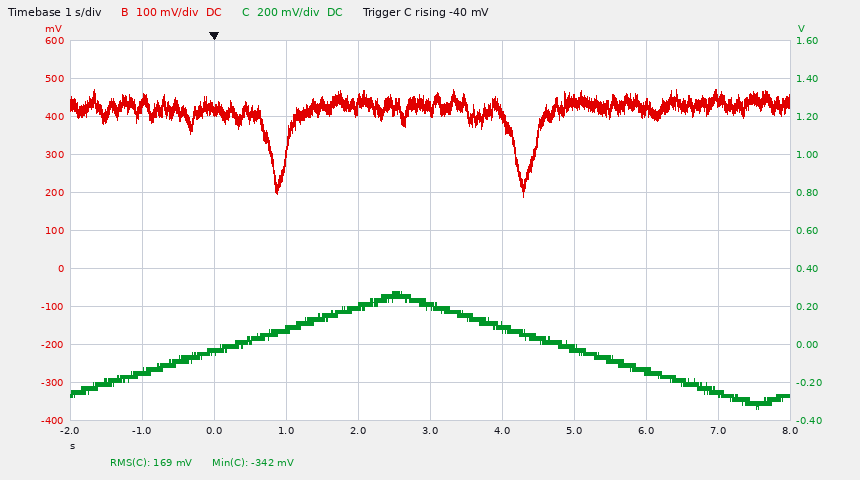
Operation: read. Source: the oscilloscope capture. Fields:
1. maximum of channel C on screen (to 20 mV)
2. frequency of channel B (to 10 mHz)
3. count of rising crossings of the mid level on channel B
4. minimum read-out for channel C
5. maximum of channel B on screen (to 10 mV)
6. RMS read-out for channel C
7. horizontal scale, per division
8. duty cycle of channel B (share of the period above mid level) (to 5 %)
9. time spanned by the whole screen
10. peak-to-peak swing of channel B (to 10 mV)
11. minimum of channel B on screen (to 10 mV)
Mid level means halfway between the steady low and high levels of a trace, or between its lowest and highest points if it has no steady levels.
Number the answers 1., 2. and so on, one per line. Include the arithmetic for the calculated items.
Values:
1. 280 mV
2. 290 mHz
3. 2
4. -342 mV
5. 470 mV
6. 169 mV
7. 1 s
8. 90 %
9. 10 s
10. 470 mV − (190 mV) = 280 mV
11. 190 mV
